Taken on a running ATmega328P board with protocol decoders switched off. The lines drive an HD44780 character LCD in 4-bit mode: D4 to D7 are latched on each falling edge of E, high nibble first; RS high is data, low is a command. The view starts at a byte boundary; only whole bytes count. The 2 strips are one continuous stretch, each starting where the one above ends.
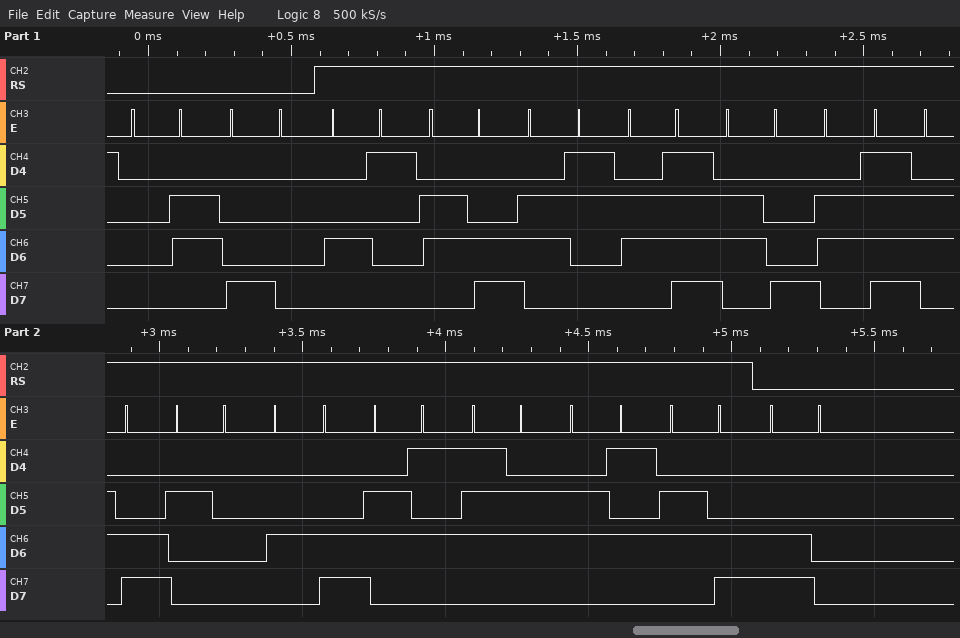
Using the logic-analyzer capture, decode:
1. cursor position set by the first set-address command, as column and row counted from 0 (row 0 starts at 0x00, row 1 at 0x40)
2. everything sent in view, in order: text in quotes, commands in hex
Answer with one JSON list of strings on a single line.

["column 0, row 0", "0x06 0x80 \"Alcohol Level\" 0xC0"]
